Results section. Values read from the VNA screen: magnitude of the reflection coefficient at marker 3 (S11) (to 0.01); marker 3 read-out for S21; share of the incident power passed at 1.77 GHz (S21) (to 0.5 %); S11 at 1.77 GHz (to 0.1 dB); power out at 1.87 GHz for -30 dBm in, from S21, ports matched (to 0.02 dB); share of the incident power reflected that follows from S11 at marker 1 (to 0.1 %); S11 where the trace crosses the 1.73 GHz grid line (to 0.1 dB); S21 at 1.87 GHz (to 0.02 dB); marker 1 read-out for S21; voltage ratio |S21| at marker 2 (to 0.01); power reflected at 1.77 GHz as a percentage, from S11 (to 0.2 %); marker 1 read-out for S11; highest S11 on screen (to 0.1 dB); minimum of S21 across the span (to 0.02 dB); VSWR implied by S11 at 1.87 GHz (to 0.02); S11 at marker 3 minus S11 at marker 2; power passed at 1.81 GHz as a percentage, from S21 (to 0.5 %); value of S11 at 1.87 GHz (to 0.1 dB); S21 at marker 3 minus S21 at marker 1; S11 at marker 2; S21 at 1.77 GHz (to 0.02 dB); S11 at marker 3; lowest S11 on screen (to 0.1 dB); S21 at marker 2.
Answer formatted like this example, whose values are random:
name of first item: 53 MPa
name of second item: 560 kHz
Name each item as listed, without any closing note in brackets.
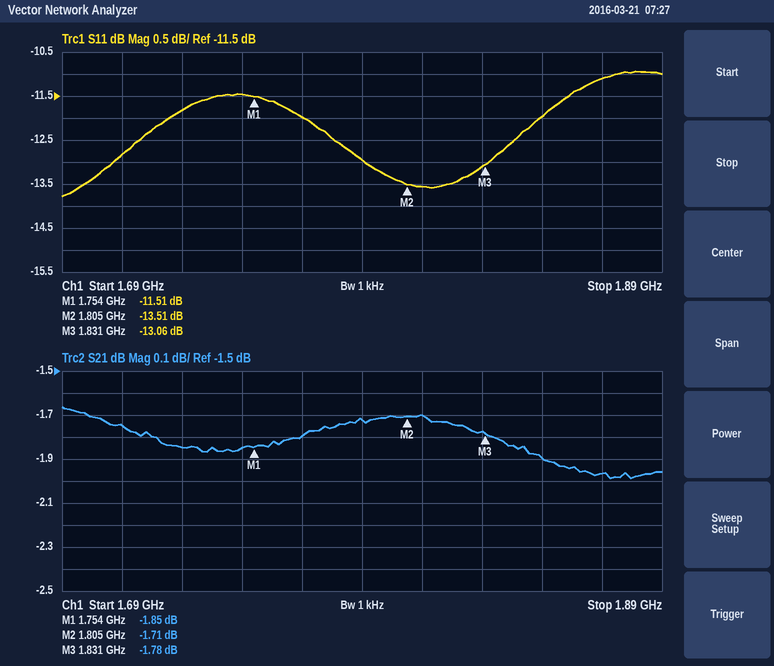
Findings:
magnitude of the reflection coefficient at marker 3 (S11): 0.22
marker 3 read-out for S21: -1.78 dB
share of the incident power passed at 1.77 GHz (S21): 66.0 %
S11 at 1.77 GHz: -12.0 dB
power out at 1.87 GHz for -30 dBm in, from S21, ports matched: -31.96 dBm
share of the incident power reflected that follows from S11 at marker 1: 7.1 %
S11 where the trace crosses the 1.73 GHz grid line: -11.8 dB
S21 at 1.87 GHz: -1.96 dB
marker 1 read-out for S21: -1.85 dB
voltage ratio |S21| at marker 2: 0.82
power reflected at 1.77 GHz as a percentage, from S11: 6.4 %
marker 1 read-out for S11: -11.51 dB
highest S11 on screen: -10.9 dB
minimum of S21 across the span: -1.98 dB
VSWR implied by S11 at 1.87 GHz: 1.78
S11 at marker 3 minus S11 at marker 2: 0.45 dB
power passed at 1.81 GHz as a percentage, from S21: 67.5 %
value of S11 at 1.87 GHz: -11.1 dB
S21 at marker 3 minus S21 at marker 1: 0.07 dB
S11 at marker 2: -13.51 dB
S21 at 1.77 GHz: -1.80 dB
S11 at marker 3: -13.06 dB
lowest S11 on screen: -13.8 dB
S21 at marker 2: -1.71 dB
